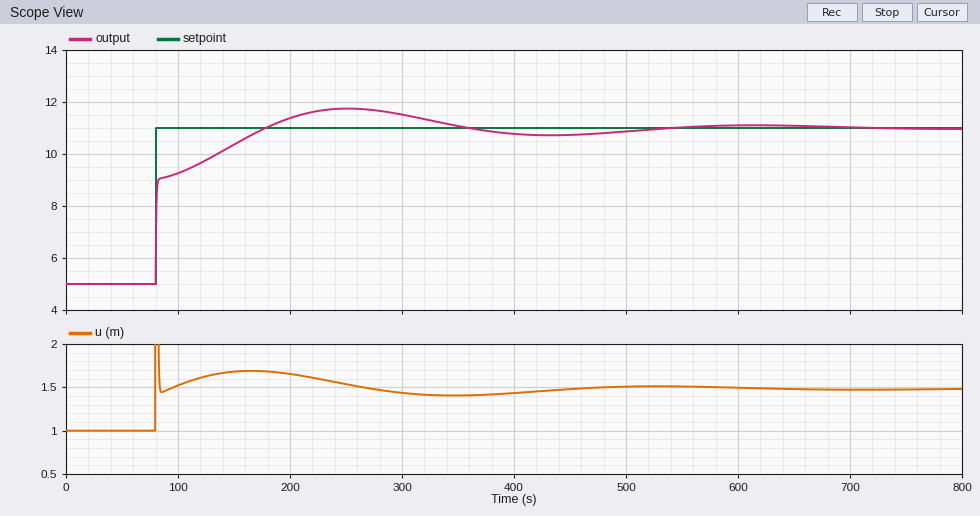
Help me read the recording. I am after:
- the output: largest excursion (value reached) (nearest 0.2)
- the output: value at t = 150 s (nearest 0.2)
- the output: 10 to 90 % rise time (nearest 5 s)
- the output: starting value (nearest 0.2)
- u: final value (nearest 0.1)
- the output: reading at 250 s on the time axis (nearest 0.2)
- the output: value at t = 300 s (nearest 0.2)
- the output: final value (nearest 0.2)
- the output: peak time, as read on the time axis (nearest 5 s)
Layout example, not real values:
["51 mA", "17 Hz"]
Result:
["11.8", "10.4", "70 s", "5.0", "1.5", "11.8", "11.6", "11.0", "250 s"]
